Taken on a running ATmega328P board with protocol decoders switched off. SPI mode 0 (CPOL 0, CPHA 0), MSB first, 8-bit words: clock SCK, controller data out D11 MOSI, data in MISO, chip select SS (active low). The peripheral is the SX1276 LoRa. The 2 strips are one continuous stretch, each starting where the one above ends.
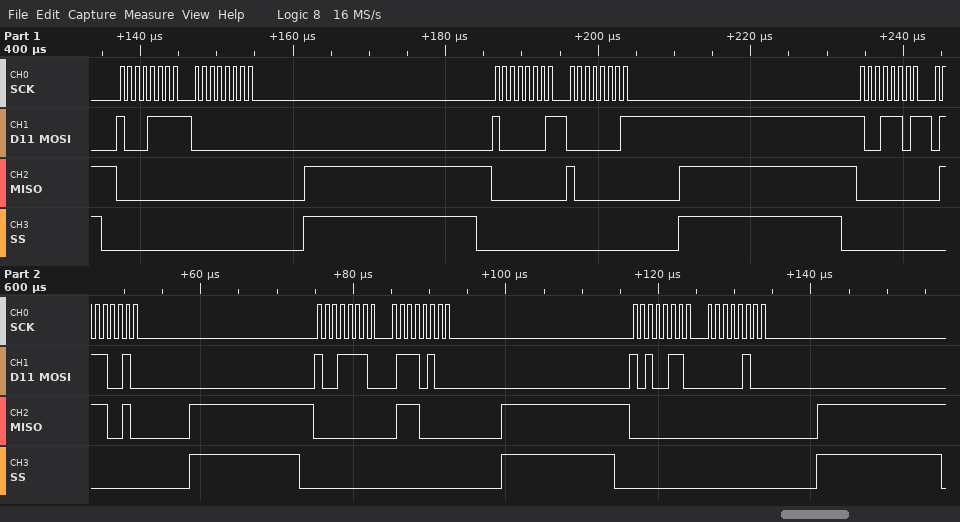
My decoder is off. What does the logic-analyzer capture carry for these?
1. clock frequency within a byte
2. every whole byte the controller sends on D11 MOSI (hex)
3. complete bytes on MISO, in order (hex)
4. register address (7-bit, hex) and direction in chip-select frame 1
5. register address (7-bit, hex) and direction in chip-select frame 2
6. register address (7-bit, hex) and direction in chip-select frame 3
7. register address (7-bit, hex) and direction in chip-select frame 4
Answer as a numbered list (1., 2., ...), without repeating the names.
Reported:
1. 1 MHz
2. 0x8F 0x00 0x81 0x01 0x9D 0x72 0x9E 0x74 0xA6 0x04
3. 0x00 0x00 0x00 0x80 0x00 0x72 0x00 0x70 0x00 0x00
4. 0x0F write
5. 0x01 write
6. 0x1D write
7. 0x1E write
